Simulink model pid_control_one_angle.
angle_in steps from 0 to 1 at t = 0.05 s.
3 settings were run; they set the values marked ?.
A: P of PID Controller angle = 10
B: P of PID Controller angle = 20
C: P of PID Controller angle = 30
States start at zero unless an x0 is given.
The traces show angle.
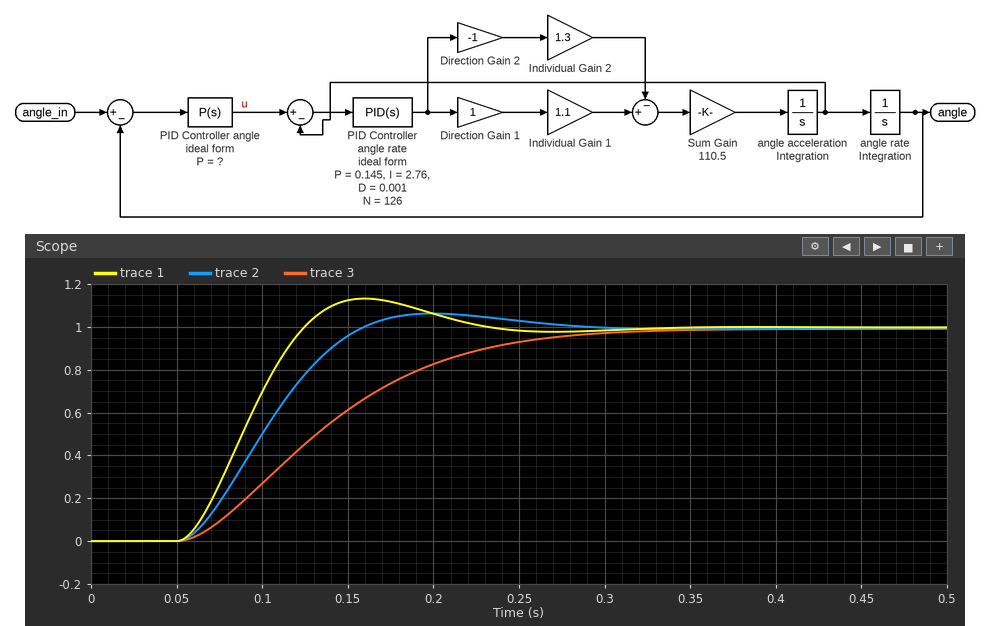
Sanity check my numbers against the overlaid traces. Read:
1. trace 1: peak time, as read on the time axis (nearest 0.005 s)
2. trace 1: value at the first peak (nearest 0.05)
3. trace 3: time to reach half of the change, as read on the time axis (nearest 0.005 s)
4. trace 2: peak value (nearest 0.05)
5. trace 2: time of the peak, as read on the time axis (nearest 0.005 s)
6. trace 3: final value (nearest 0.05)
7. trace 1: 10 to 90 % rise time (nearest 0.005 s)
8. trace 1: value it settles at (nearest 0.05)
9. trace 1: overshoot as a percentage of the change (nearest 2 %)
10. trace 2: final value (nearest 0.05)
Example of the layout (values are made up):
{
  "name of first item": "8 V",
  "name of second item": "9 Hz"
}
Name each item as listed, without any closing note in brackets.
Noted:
{
  "trace 1: peak time, as read on the time axis": "0.160 s",
  "trace 1: value at the first peak": "1.15",
  "trace 3: time to reach half of the change, as read on the time axis": "0.130 s",
  "trace 2: peak value": "1.05",
  "trace 2: time of the peak, as read on the time axis": "0.200 s",
  "trace 3: final value": "1.00",
  "trace 1: 10 to 90 % rise time": "0.050 s",
  "trace 1: value it settles at": "1.00",
  "trace 1: overshoot as a percentage of the change": "14 %",
  "trace 2: final value": "1.00"
}
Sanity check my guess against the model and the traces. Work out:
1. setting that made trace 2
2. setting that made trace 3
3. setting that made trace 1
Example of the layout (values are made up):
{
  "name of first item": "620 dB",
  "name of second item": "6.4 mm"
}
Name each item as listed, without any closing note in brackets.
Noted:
{
  "setting that made trace 2": "B",
  "setting that made trace 3": "A",
  "setting that made trace 1": "C"
}
